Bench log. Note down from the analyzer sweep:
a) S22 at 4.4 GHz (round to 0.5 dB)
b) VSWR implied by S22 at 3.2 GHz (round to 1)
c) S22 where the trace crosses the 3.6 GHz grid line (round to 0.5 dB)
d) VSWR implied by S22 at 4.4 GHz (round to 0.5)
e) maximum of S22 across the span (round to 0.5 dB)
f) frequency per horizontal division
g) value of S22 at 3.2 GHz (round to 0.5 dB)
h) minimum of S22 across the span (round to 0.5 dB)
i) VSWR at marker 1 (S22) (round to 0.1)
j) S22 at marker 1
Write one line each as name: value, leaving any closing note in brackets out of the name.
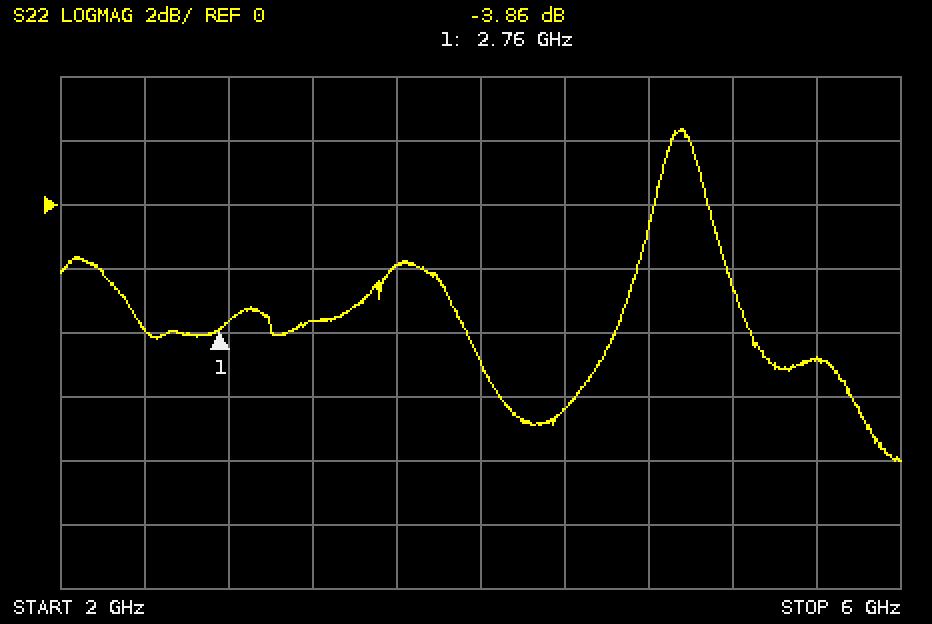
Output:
S22 at 4.4 GHz: -6.5 dB
VSWR implied by S22 at 3.2 GHz: 5
S22 where the trace crosses the 3.6 GHz grid line: -2.0 dB
VSWR implied by S22 at 4.4 GHz: 3.0
maximum of S22 across the span: 2.5 dB
frequency per horizontal division: 400 MHz
value of S22 at 3.2 GHz: -3.5 dB
minimum of S22 across the span: -8.0 dB
VSWR at marker 1 (S22): 4.6
S22 at marker 1: -3.86 dB
